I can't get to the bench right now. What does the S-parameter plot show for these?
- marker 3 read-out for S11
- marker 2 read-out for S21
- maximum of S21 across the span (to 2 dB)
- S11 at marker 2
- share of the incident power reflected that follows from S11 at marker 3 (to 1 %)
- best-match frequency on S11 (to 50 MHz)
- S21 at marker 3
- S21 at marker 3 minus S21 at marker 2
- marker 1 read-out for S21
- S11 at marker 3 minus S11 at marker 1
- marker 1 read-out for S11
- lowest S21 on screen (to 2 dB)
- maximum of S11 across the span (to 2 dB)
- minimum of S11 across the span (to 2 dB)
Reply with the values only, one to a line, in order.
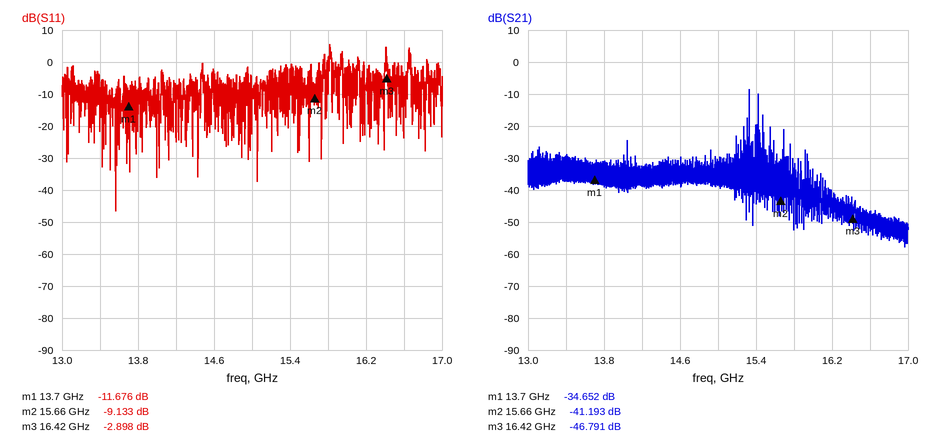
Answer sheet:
-2.898 dB
-41.193 dB
-8 dB
-9.133 dB
51 %
13.55 GHz
-46.791 dB
-5.598 dB
-34.652 dB
8.778 dB
-11.676 dB
-58 dB
6 dB
-46 dB
